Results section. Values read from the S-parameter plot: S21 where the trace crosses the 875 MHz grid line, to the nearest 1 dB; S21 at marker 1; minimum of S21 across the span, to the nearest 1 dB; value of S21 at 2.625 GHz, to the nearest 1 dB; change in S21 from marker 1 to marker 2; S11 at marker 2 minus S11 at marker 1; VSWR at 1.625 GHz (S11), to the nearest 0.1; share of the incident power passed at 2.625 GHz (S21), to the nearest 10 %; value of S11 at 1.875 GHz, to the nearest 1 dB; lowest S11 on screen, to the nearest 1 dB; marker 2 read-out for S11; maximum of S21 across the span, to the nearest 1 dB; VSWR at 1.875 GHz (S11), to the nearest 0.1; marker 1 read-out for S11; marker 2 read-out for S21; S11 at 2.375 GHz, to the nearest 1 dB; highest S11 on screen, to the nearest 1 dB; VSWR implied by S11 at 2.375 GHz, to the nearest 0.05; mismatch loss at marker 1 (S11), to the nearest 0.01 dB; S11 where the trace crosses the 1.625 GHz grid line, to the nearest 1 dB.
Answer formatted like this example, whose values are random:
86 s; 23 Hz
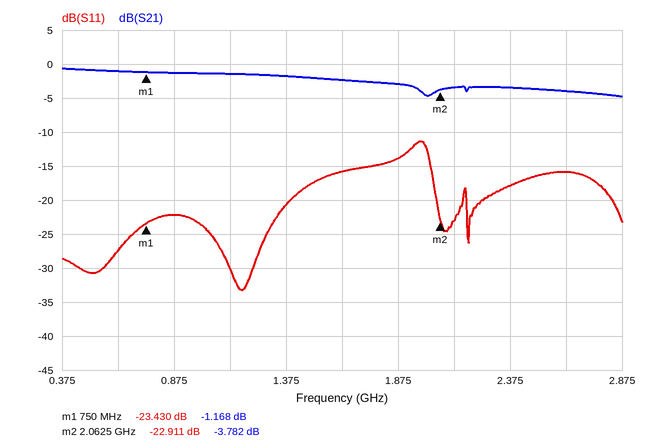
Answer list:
-1 dB; -1.168 dB; -5 dB; -4 dB; -2.614 dB; 0.519 dB; 1.4; 40 %; -14 dB; -33 dB; -22.911 dB; -1 dB; 1.5; -23.430 dB; -3.782 dB; -18 dB; -11 dB; 1.30; 0.02 dB; -16 dB
